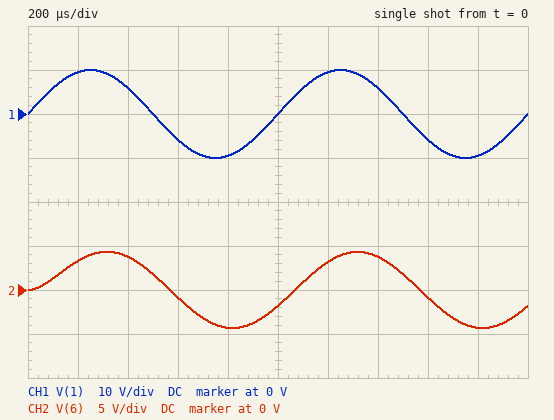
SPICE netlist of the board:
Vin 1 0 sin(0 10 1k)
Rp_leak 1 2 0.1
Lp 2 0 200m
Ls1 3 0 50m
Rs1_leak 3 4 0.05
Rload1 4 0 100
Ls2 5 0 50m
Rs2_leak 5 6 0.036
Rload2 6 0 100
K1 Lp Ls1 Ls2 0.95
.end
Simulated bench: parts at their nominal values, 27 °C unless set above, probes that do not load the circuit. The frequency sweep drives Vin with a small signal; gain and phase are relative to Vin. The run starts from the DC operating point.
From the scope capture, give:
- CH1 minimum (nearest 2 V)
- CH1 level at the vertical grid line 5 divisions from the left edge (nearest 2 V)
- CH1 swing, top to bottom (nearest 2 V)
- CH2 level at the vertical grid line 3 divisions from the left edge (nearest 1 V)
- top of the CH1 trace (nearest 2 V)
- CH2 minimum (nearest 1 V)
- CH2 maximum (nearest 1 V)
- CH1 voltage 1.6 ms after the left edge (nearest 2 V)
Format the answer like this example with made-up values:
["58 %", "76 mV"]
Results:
["-10 V", "0 V", "20 V", "-1 V", "10 V", "-4 V", "4 V", "-6 V"]
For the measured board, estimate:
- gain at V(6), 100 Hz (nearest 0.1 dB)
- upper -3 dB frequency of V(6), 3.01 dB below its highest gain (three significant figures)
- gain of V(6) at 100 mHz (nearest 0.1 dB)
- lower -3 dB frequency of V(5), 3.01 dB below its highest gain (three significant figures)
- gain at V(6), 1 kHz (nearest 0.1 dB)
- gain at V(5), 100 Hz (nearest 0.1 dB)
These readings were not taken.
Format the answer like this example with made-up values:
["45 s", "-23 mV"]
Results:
["-6.5 dB", "2.20 kHz", "-8.6 dB", "79.5 mHz", "-7.3 dB", "-6.5 dB"]
